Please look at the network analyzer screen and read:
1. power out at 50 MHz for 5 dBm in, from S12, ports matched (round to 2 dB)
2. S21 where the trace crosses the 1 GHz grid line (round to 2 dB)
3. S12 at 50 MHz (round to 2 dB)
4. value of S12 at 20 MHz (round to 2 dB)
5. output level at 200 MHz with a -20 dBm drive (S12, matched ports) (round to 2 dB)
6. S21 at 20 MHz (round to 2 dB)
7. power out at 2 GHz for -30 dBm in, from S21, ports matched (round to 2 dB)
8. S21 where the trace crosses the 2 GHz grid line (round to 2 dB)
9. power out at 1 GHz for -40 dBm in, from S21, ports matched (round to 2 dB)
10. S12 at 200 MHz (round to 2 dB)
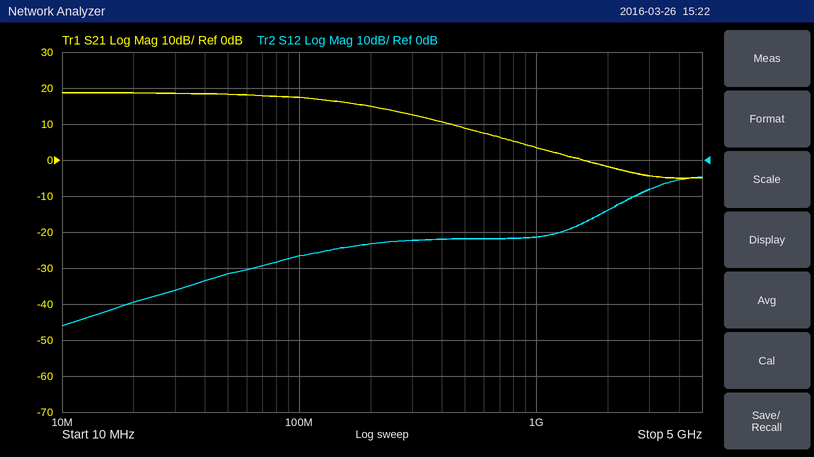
-26 dBm
4 dB
-32 dB
-40 dB
-44 dBm
18 dB
-32 dBm
-2 dB
-36 dBm
-24 dB
